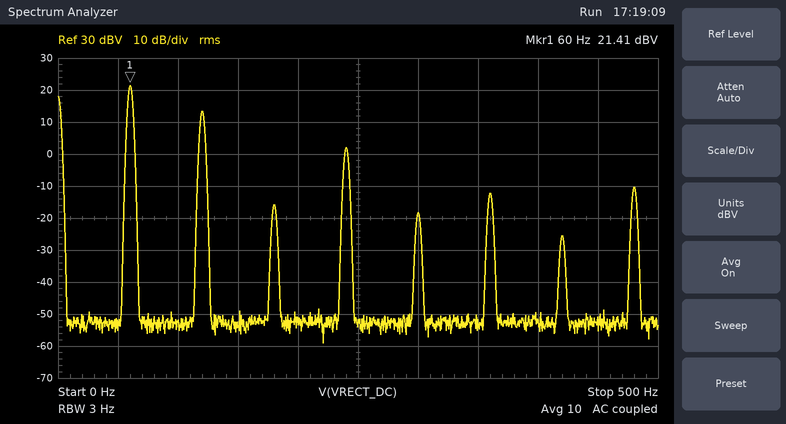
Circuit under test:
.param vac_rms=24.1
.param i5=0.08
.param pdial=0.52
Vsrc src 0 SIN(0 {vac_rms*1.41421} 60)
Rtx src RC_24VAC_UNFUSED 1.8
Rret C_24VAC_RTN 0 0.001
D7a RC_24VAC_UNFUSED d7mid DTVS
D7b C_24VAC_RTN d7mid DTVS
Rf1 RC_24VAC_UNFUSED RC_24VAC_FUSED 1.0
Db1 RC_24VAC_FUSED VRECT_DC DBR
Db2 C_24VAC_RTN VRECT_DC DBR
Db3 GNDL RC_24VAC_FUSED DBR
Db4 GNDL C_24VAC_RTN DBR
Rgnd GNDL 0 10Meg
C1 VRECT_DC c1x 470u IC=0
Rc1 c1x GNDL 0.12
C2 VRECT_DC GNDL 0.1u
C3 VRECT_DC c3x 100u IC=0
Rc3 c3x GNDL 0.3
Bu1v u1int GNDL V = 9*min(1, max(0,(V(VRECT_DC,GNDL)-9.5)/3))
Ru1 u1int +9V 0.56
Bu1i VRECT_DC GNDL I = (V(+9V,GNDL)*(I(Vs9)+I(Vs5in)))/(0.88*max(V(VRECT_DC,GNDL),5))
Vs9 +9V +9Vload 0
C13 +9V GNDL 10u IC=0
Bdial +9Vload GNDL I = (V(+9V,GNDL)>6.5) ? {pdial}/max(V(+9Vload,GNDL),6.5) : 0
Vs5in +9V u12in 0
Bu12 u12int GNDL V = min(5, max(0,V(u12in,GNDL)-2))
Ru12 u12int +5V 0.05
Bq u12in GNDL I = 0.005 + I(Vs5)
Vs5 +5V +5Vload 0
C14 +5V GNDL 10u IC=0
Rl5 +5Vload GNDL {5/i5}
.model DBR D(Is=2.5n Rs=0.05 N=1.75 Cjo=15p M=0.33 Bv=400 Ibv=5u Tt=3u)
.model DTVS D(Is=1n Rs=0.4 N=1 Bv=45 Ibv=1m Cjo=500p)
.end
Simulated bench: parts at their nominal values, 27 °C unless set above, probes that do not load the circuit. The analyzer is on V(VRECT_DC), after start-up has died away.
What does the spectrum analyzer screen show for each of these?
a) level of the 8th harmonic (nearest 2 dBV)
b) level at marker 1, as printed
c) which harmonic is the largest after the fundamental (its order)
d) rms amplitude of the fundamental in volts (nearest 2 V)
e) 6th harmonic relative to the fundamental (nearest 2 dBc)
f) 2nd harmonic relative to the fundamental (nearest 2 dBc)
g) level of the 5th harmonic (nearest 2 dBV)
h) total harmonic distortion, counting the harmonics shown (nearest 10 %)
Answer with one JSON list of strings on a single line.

["-10 dBV", "21.41 dBV", "2", "12 V", "-34 dBc", "-8 dBc", "-18 dBV", "40 %"]
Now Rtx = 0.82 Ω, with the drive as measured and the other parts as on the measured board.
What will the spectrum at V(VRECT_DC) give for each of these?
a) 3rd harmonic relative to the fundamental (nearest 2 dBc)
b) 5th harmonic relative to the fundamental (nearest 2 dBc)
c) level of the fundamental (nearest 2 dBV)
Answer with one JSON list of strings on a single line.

["-36 dBc", "-42 dBc", "22 dBV"]
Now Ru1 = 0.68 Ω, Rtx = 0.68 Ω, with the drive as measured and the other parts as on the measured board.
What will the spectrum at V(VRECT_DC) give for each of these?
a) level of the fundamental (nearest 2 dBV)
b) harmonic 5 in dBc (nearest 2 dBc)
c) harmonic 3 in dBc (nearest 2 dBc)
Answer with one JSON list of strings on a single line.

["22 dBV", "-42 dBc", "-36 dBc"]
